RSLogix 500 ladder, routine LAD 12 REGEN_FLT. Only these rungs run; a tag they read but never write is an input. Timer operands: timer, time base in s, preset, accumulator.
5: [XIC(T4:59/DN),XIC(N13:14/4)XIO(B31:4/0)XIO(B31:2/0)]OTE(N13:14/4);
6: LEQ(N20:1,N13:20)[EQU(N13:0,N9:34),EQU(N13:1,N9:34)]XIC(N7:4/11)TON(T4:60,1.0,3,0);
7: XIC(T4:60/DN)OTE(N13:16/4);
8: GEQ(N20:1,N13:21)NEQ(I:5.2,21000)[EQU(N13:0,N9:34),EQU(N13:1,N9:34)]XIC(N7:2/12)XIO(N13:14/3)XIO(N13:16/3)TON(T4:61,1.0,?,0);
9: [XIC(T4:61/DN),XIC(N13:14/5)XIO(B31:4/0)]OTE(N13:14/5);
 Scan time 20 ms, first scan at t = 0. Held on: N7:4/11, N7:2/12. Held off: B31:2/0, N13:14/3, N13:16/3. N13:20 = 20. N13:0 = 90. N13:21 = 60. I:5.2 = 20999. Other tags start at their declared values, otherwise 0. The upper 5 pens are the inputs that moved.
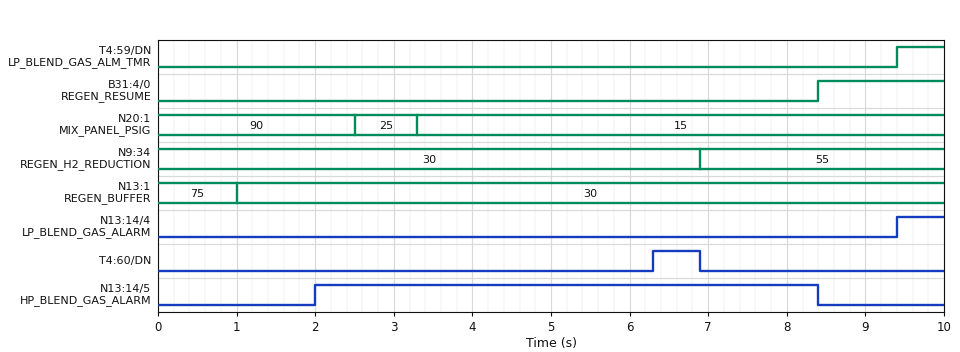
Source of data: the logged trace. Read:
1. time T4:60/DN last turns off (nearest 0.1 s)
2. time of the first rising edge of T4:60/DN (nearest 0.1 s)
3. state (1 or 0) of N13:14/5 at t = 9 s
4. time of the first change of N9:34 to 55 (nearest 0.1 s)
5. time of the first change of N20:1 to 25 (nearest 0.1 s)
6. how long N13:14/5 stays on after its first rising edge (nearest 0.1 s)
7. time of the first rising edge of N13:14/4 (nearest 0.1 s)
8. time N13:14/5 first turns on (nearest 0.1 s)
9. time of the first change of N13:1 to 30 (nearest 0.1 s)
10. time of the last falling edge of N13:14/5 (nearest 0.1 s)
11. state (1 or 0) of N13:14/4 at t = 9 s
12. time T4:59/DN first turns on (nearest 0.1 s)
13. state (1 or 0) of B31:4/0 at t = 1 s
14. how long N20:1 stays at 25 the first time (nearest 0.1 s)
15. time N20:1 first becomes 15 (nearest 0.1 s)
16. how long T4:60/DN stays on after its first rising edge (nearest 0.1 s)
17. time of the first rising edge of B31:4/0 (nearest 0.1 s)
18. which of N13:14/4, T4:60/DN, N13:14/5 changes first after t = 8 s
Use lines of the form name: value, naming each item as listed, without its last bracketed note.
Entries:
time T4:60/DN last turns off: 6.9 s
time of the first rising edge of T4:60/DN: 6.3 s
state (1 or 0) of N13:14/5 at t = 9 s: 0
time of the first change of N9:34 to 55: 6.9 s
time of the first change of N20:1 to 25: 2.5 s
how long N13:14/5 stays on after its first rising edge: 6.4 s
time of the first rising edge of N13:14/4: 9.4 s
time N13:14/5 first turns on: 2.0 s
time of the first change of N13:1 to 30: 1.0 s
time of the last falling edge of N13:14/5: 8.4 s
state (1 or 0) of N13:14/4 at t = 9 s: 0
time T4:59/DN first turns on: 9.4 s
state (1 or 0) of B31:4/0 at t = 1 s: 0
how long N20:1 stays at 25 the first time: 0.8 s
time N20:1 first becomes 15: 3.3 s
how long T4:60/DN stays on after its first rising edge: 0.6 s
time of the first rising edge of B31:4/0: 8.4 s
which of N13:14/4, T4:60/DN, N13:14/5 changes first after t = 8 s: N13:14/5
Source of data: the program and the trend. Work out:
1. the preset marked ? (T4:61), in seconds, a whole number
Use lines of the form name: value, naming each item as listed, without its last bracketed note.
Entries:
the preset marked ? (T4:61), in seconds, a whole number: 1 s
